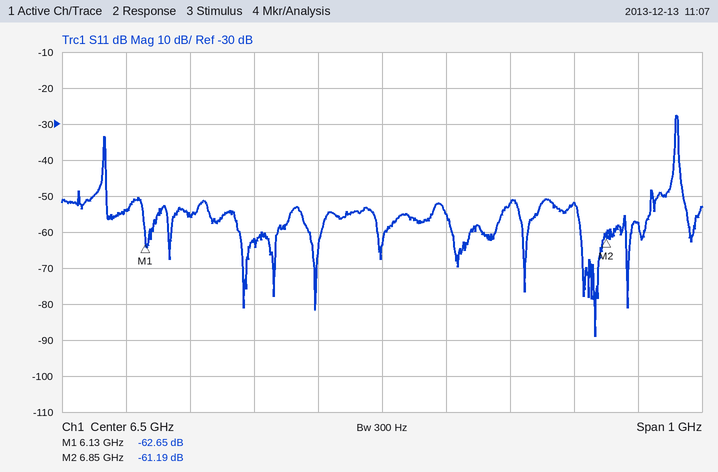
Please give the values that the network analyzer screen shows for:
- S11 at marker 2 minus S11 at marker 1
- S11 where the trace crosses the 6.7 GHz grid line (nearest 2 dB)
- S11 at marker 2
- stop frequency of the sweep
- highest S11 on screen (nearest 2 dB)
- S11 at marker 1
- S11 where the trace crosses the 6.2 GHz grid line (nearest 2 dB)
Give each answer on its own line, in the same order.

1.46 dB
-52 dB
-61.19 dB
7 GHz
-28 dB
-62.65 dB
-56 dB
